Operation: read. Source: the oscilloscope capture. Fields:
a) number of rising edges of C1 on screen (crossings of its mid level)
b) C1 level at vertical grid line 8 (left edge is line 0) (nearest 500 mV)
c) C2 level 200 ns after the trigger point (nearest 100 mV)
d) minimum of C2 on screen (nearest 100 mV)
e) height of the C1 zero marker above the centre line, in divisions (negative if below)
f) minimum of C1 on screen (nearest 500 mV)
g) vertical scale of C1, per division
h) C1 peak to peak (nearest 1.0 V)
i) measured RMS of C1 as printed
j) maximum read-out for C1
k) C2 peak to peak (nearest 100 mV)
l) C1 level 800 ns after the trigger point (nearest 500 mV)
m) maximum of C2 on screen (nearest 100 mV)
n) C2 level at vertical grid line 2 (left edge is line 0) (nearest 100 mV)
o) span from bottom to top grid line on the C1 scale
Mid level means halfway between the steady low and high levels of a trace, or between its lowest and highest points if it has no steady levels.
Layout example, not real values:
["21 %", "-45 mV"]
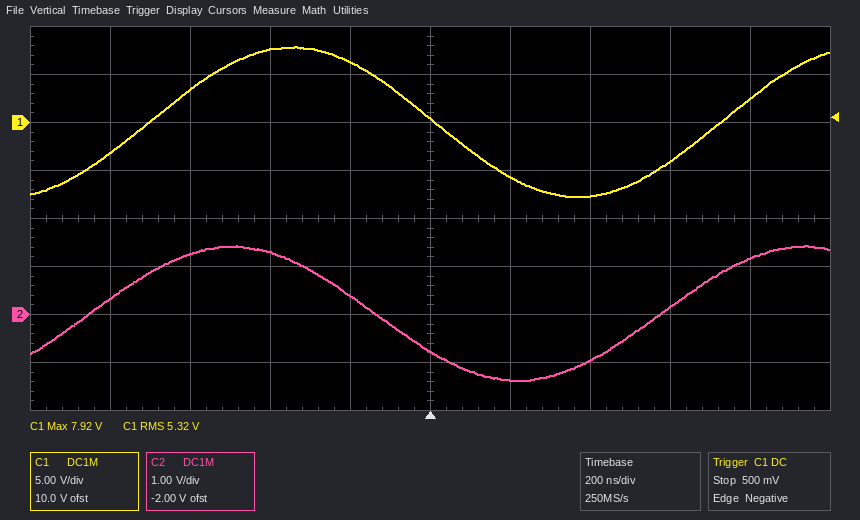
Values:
["2", "-4.0 V", "-1.4 V", "-1.4 V", "+2.0 div", "-7.5 V", "5 V", "16.0 V", "5.32 V", "7.92 V", "2.8 V", "2.5 V", "1.4 V", "1.3 V", "40 V"]
